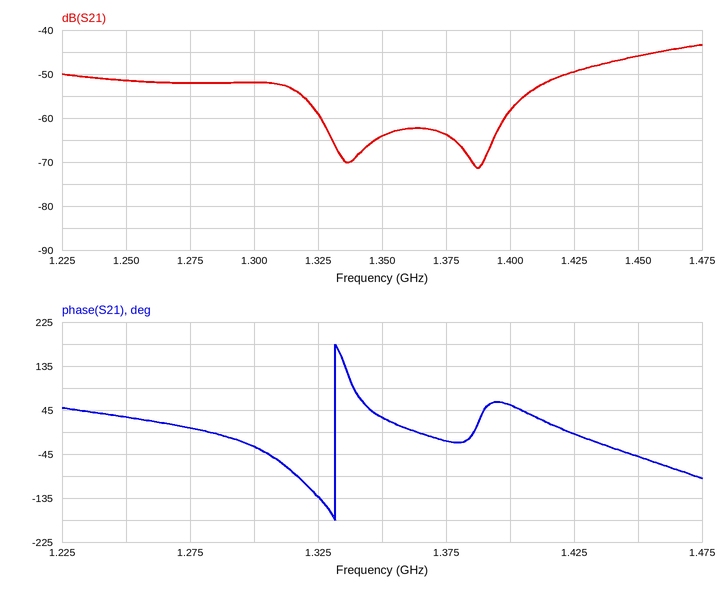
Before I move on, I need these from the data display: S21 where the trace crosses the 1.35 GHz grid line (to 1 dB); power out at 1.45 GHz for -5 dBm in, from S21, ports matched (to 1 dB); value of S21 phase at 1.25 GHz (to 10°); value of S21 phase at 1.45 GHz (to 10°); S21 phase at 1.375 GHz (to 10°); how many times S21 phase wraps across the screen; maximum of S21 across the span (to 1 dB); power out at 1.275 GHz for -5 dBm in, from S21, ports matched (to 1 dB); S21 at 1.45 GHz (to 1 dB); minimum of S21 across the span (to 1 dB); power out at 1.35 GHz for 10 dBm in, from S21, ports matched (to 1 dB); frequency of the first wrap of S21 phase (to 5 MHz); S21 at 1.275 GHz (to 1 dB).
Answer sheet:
-64 dB
-51 dBm
30°
-50°
-20°
1
-43 dB
-57 dBm
-46 dB
-71 dB
-54 dBm
1.330 GHz
-52 dB
